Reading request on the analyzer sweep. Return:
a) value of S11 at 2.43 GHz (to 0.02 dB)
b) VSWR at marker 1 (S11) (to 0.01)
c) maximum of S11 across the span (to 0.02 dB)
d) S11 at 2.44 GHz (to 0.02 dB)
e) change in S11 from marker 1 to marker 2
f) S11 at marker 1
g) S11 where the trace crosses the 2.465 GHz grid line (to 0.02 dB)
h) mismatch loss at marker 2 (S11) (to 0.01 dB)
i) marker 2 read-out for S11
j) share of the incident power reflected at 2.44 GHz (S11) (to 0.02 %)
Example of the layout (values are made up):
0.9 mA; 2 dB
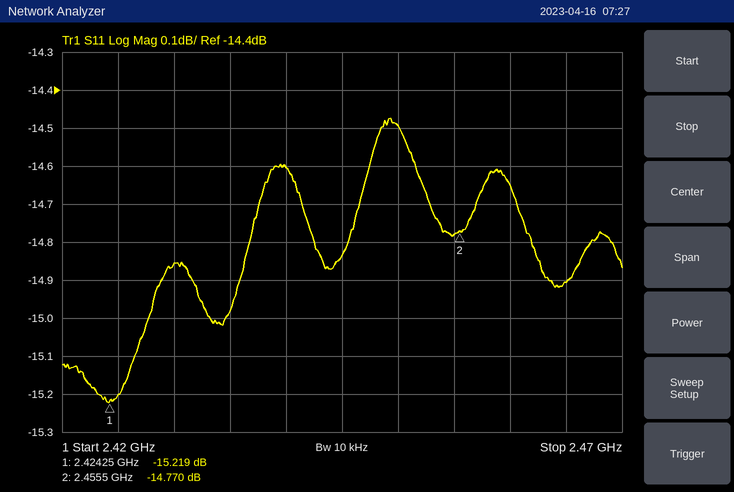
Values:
-14.86 dB; 1.42; -14.48 dB; -14.60 dB; 0.449 dB; -15.219 dB; -14.90 dB; 0.15 dB; -14.770 dB; 3.46 %
